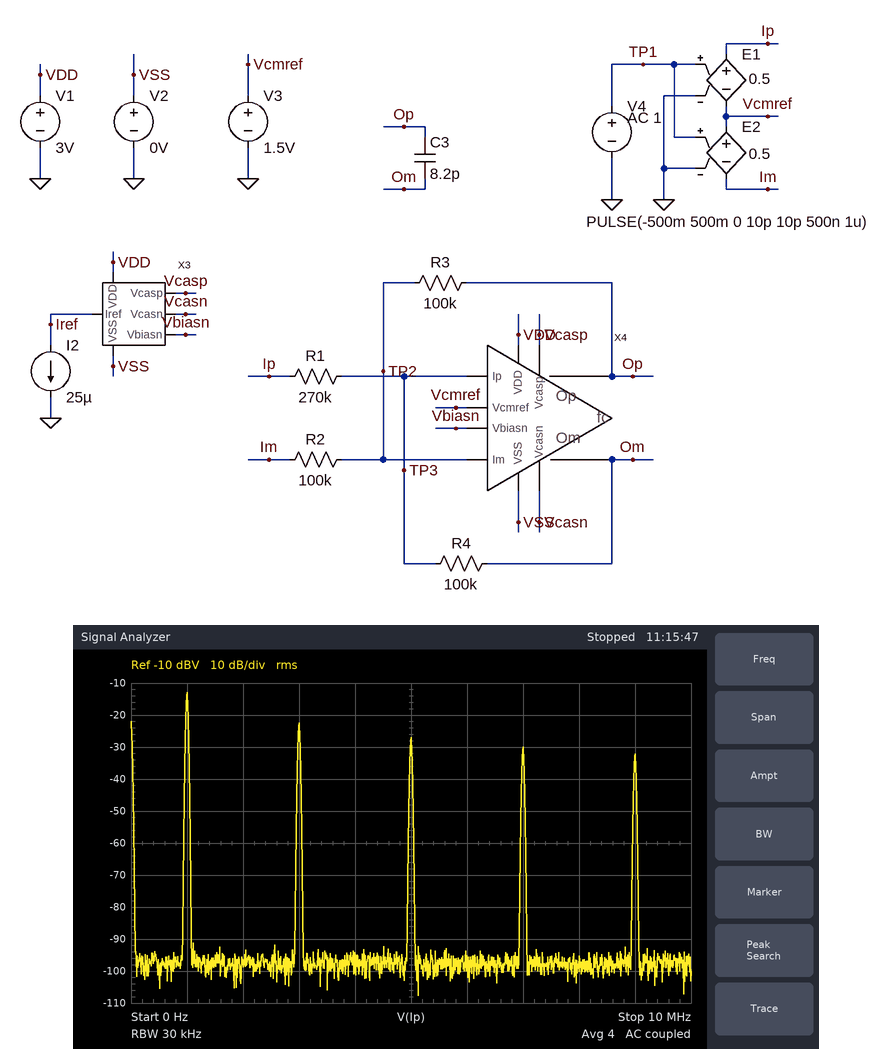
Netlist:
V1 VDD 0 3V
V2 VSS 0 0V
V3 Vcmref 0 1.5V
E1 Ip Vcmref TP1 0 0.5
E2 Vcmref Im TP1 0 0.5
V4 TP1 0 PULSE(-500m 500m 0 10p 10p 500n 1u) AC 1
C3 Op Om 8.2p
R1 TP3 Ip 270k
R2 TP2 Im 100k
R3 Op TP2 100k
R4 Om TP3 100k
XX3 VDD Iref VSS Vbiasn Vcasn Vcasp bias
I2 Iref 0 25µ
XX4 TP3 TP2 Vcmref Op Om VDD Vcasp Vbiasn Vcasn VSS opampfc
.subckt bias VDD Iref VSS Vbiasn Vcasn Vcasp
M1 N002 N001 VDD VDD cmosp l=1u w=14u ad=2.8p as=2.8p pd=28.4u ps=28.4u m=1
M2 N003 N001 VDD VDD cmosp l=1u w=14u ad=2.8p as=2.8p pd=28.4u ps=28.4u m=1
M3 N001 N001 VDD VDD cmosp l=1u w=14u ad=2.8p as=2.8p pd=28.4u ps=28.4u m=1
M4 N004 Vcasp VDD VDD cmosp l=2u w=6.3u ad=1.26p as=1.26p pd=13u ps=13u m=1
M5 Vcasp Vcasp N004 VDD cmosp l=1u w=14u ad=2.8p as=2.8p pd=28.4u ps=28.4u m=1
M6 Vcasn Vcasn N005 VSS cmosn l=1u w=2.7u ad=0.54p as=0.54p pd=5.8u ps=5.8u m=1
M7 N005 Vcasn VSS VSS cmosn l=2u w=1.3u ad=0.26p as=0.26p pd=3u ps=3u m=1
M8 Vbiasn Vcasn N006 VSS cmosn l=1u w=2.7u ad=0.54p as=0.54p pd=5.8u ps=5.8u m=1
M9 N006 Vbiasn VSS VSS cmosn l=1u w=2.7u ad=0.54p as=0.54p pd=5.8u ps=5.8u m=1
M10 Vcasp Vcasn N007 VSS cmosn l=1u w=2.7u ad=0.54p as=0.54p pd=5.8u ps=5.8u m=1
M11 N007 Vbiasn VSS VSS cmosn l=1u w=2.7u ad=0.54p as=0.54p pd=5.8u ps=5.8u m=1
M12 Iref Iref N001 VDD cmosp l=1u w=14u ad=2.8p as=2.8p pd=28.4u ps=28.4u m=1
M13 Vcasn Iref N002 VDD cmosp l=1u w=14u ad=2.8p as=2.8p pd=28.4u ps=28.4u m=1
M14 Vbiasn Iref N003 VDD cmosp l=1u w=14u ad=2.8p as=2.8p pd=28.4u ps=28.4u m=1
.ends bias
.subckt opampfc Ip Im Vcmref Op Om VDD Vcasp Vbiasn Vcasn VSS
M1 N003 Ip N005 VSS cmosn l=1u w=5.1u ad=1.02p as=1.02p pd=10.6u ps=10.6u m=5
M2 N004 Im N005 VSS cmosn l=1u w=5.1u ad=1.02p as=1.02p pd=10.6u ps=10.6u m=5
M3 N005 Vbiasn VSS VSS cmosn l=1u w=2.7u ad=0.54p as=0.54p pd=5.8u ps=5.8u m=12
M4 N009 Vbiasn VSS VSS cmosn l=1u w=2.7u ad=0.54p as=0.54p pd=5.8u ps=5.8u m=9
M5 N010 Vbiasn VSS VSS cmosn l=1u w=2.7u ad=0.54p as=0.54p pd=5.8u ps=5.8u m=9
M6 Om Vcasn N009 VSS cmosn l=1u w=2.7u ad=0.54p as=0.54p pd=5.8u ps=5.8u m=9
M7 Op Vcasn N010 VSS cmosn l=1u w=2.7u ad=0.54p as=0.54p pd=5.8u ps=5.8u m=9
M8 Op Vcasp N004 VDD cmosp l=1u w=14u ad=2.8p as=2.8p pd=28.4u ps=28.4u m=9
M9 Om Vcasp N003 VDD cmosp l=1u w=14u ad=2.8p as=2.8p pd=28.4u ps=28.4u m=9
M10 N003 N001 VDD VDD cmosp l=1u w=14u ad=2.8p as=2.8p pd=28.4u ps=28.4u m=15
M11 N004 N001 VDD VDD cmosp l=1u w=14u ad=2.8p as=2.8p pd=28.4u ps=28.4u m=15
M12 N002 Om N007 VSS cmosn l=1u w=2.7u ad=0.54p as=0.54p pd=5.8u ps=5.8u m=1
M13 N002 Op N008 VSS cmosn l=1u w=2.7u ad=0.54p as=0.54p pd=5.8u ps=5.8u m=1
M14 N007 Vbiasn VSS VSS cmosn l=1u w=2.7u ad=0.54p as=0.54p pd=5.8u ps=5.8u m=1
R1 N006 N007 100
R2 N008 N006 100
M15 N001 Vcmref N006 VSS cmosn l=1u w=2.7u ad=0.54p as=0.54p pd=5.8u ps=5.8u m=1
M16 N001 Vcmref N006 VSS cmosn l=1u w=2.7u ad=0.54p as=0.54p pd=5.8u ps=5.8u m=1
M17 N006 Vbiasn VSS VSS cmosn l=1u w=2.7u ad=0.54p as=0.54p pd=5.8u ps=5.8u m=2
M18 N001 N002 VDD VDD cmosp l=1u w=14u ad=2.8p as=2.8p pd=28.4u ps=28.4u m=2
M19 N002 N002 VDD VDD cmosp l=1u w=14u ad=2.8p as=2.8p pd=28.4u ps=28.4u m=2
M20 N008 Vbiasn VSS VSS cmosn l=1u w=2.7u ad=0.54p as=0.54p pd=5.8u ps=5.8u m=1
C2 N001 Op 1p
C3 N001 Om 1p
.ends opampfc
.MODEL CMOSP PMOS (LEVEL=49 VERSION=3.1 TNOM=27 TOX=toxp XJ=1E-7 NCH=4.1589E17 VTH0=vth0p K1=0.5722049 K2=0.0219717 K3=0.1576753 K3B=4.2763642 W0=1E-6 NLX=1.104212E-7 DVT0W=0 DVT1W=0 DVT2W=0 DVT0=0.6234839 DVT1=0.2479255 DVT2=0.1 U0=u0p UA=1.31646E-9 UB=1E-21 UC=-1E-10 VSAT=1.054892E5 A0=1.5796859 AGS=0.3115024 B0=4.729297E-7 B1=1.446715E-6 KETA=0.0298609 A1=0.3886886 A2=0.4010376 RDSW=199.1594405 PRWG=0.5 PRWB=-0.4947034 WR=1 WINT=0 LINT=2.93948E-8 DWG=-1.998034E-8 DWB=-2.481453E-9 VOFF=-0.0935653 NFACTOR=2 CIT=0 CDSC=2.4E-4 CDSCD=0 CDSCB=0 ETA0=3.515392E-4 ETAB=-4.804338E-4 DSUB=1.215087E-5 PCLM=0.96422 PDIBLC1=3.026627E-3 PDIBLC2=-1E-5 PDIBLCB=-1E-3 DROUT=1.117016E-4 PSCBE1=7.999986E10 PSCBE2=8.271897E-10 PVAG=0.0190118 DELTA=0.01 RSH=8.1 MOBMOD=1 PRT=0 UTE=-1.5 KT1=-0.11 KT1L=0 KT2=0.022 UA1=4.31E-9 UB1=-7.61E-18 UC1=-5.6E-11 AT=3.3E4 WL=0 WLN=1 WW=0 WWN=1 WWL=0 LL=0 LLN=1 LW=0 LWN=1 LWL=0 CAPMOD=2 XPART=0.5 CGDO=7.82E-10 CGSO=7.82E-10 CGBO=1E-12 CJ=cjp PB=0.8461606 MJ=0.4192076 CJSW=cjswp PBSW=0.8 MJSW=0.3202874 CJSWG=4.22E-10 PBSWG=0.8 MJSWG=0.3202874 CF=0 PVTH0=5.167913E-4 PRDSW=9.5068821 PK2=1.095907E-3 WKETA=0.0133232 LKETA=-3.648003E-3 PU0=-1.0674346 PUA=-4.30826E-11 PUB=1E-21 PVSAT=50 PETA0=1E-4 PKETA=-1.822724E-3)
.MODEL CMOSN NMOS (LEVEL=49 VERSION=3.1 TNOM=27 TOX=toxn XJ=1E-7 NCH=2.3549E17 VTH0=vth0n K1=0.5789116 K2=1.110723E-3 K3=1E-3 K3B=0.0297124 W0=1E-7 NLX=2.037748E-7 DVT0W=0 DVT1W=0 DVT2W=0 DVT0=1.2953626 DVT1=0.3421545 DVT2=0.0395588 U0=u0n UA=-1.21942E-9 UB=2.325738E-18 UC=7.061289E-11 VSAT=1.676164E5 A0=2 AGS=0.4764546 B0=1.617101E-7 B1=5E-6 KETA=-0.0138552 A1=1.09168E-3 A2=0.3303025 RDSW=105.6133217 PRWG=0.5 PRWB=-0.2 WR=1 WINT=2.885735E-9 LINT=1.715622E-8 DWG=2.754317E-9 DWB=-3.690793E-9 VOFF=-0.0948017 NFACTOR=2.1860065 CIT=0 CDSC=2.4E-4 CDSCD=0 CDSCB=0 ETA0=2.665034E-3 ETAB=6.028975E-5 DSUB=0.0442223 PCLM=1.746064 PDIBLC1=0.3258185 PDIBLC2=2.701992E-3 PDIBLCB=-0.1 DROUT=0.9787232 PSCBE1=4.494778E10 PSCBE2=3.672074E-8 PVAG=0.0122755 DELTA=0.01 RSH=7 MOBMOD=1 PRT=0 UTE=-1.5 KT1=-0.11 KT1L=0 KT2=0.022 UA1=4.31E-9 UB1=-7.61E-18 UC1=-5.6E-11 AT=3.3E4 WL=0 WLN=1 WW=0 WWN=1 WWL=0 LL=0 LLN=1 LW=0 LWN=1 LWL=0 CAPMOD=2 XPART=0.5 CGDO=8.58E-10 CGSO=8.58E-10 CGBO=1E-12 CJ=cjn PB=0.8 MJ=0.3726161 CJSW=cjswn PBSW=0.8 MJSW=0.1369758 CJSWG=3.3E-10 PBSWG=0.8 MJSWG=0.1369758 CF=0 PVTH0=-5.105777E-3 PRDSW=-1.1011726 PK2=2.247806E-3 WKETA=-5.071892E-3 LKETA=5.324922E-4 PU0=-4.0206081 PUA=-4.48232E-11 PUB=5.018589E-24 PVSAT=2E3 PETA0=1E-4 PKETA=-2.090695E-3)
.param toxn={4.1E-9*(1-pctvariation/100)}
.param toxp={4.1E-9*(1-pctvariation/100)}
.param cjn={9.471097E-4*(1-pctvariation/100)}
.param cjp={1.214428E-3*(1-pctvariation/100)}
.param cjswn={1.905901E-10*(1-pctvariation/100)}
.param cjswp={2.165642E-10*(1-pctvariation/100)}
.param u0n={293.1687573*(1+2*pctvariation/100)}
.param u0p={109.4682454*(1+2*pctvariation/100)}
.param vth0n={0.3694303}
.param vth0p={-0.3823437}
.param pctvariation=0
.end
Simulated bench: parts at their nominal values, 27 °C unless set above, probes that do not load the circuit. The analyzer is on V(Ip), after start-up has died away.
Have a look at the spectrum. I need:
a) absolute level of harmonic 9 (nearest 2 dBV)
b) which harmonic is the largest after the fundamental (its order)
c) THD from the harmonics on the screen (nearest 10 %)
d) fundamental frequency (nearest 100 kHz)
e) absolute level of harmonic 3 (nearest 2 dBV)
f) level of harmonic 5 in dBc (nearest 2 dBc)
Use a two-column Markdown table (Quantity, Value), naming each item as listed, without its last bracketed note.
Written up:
| Quantity | Value |
|---|---|
| absolute level of harmonic 9 | -32 dBV |
| which harmonic is the largest after the fundamental | 3 |
| THD from the harmonics on the screen | 40 % |
| fundamental frequency | 1.0 MHz |
| absolute level of harmonic 3 | -22 dBV |
| level of harmonic 5 in dBc | -14 dBc |
